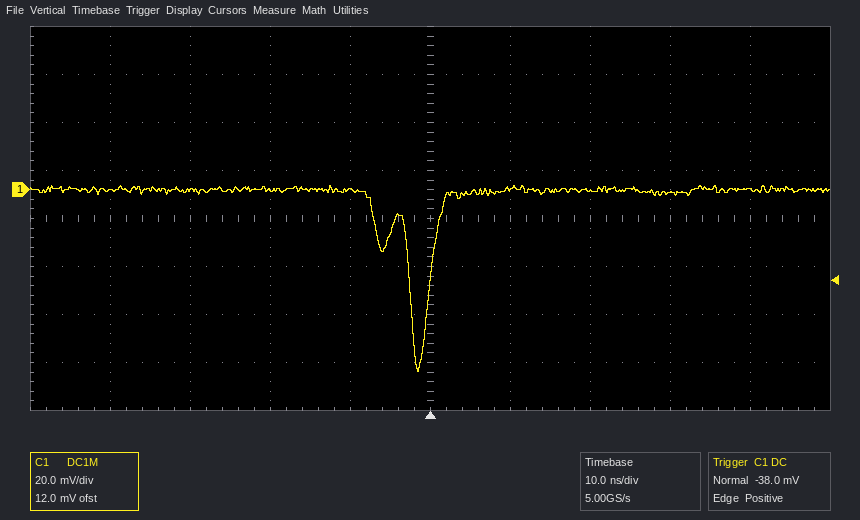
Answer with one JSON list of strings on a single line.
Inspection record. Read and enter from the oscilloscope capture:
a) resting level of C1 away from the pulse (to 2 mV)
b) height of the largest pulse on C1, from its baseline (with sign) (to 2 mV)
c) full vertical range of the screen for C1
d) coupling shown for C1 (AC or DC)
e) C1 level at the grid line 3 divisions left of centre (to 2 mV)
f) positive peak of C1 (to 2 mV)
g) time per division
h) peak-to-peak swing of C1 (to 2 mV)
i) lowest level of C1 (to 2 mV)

["0 mV", "-76 mV", "160 mV", "DC", "0 mV", "2 mV", "10 ns", "78 mV", "-76 mV"]
